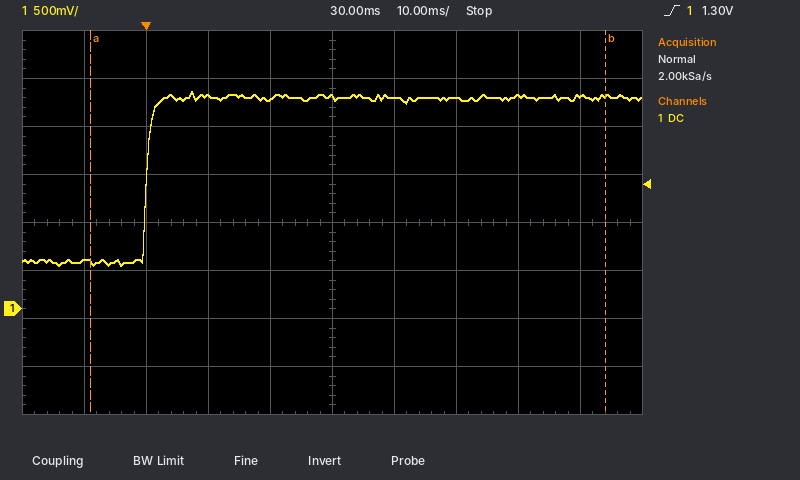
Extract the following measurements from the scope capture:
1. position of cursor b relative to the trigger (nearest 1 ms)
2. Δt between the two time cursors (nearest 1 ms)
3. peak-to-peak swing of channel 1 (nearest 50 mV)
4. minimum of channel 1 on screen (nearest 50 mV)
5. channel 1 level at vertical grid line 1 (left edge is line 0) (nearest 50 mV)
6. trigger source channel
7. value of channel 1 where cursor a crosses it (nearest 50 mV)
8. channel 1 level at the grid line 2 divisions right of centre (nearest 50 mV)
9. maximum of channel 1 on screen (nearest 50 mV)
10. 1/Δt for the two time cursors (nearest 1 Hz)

+74 ms
83 ms
1.80 V
450 mV
500 mV
channel 1
500 mV
2.20 V
2.25 V
12 Hz
